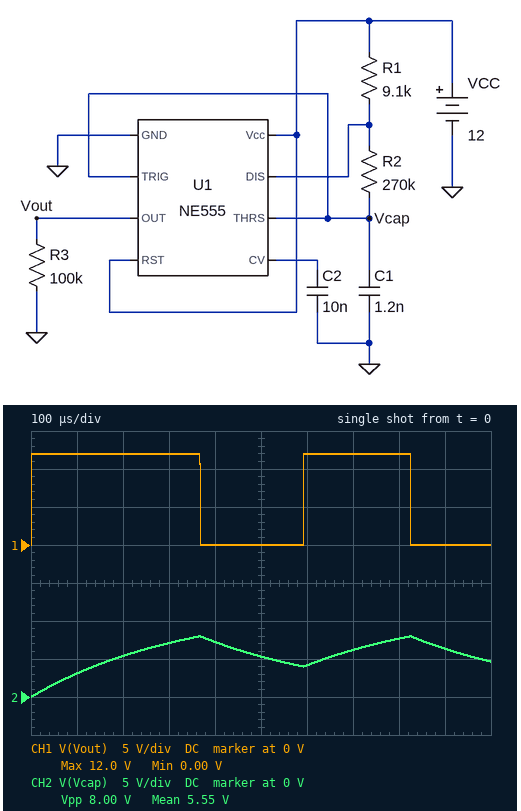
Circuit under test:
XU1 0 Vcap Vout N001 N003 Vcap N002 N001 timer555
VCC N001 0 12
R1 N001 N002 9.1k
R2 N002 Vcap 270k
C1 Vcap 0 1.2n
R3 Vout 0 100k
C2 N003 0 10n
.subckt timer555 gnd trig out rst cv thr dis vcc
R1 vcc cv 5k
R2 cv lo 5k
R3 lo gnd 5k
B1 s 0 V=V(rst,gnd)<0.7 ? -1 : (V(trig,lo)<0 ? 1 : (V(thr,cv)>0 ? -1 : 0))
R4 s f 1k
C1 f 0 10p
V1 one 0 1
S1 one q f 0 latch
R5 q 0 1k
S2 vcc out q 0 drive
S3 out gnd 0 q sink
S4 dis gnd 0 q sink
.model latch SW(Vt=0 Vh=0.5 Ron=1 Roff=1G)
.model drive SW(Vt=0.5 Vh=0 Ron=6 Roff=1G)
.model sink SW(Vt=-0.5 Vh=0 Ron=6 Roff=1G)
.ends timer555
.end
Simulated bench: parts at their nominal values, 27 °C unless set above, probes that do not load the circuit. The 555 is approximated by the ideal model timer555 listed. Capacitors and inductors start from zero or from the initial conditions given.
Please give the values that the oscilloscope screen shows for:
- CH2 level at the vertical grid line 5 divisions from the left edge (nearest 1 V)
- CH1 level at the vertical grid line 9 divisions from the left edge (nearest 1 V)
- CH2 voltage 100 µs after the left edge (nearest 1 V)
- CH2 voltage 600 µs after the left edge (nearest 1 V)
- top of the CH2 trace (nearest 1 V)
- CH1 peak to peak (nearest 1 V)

5 V
0 V
3 V
4 V
8 V
12 V
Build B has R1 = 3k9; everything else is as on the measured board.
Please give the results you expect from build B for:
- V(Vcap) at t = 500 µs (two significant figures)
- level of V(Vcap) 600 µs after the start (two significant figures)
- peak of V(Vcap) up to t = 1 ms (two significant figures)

5.2 V
4.3 V
8.0 V
